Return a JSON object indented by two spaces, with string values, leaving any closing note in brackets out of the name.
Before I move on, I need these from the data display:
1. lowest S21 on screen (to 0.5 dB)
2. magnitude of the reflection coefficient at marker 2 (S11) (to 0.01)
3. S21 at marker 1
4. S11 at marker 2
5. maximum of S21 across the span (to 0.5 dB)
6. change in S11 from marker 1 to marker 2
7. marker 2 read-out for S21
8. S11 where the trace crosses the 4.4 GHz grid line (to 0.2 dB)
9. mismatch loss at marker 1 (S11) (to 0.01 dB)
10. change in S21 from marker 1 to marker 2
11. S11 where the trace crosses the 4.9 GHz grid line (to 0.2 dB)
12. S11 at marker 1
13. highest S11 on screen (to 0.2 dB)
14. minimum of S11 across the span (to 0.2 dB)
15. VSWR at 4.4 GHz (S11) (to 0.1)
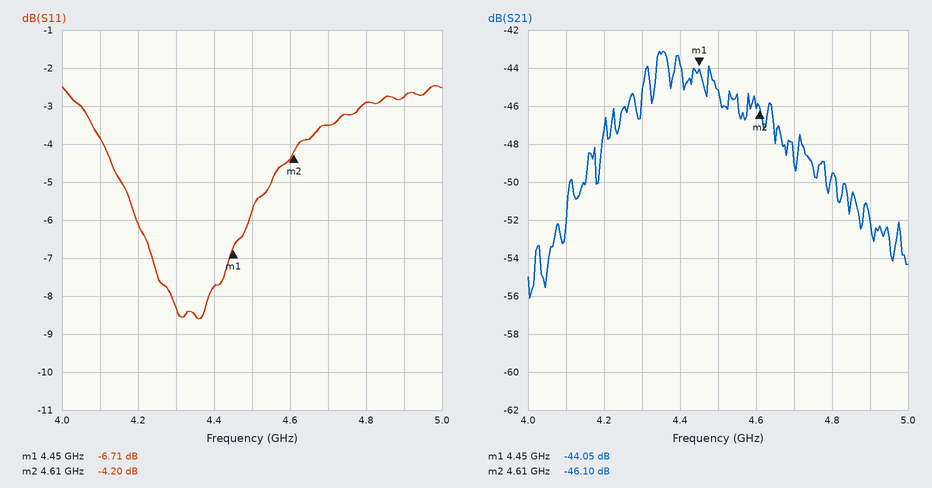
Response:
{
  "lowest S21 on screen": "-56.0 dB",
  "magnitude of the reflection coefficient at marker 2 (S11)": "0.62",
  "S21 at marker 1": "-44.05 dB",
  "S11 at marker 2": "-4.20 dB",
  "maximum of S21 across the span": "-43.0 dB",
  "change in S11 from marker 1 to marker 2": "2.51 dB",
  "marker 2 read-out for S21": "-46.10 dB",
  "S11 where the trace crosses the 4.4 GHz grid line": "-7.8 dB",
  "mismatch loss at marker 1 (S11)": "1.04 dB",
  "change in S21 from marker 1 to marker 2": "-2.05 dB",
  "S11 where the trace crosses the 4.9 GHz grid line": "-2.8 dB",
  "S11 at marker 1": "-6.71 dB",
  "highest S11 on screen": "-2.4 dB",
  "minimum of S11 across the span": "-8.6 dB",
  "VSWR at 4.4 GHz (S11)": "2.4"
}
